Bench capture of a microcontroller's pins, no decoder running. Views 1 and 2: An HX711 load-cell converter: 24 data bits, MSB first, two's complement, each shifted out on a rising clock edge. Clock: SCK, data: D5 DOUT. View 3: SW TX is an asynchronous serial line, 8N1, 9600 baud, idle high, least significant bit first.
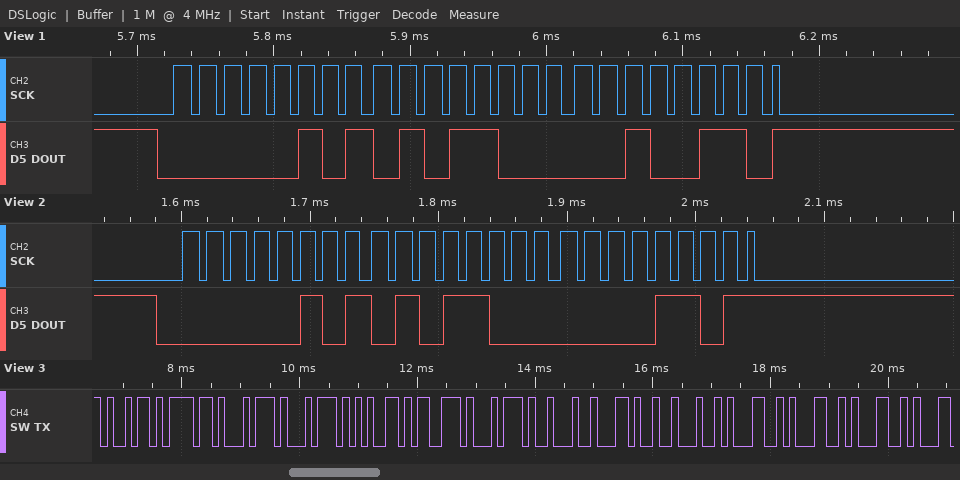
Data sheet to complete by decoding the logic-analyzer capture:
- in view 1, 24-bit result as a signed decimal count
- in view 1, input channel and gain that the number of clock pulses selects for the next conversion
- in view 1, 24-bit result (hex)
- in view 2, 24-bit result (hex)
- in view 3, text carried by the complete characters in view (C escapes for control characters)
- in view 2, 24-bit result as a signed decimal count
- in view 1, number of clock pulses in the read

350246
channel A, gain 128
0x055826
0x05580D
"iottest\",\"111"
350221
25
